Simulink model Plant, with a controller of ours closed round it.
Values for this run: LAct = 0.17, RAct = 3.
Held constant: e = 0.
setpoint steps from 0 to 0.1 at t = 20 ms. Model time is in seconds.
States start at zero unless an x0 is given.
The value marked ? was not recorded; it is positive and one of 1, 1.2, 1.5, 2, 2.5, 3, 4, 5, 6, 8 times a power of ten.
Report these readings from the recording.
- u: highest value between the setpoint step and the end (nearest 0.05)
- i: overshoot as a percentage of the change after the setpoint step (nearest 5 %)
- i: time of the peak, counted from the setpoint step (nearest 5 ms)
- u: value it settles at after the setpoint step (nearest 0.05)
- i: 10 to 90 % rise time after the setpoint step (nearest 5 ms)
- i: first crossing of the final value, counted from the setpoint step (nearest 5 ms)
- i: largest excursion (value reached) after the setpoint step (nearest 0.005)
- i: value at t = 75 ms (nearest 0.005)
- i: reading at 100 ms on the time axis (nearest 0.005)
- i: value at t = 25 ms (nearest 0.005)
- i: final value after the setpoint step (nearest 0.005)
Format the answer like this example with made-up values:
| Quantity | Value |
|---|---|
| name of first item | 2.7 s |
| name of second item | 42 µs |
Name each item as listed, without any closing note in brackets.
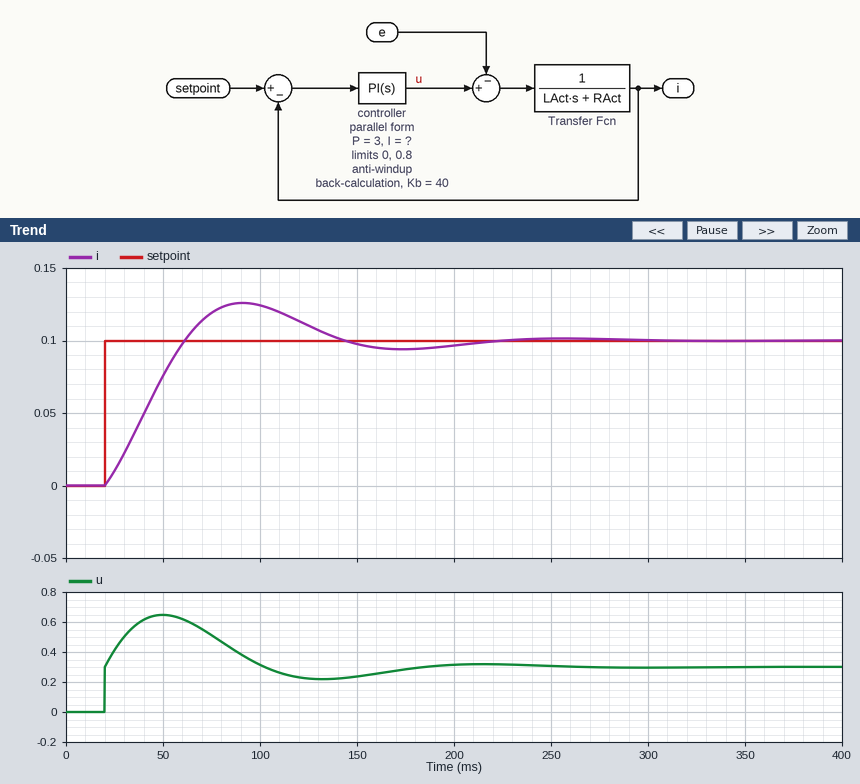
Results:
| Quantity | Value |
|---|---|
| u: highest value between the setpoint step and the end | 0.65 |
| i: overshoot as a percentage of the change after the setpoint step | 25 % |
| i: time of the peak, counted from the setpoint step | 70 ms |
| u: value it settles at after the setpoint step | 0.30 |
| i: 10 to 90 % rise time after the setpoint step | 30 ms |
| i: first crossing of the final value, counted from the setpoint step | 40 ms |
| i: largest excursion (value reached) after the setpoint step | 0.125 |
| i: value at t = 75 ms | 0.120 |
| i: reading at 100 ms on the time axis | 0.125 |
| i: value at t = 25 ms | 0.010 |
| i: final value after the setpoint step | 0.100 |
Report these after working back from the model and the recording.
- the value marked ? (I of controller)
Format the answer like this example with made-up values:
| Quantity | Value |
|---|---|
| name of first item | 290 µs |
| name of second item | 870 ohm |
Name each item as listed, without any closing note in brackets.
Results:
| Quantity | Value |
|---|---|
| the value marked ? | 300 |
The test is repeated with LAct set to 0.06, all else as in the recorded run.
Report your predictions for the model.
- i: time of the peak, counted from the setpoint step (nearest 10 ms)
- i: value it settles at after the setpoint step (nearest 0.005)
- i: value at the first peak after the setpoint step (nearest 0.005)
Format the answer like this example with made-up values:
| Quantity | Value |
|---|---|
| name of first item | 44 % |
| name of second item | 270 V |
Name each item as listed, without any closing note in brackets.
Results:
| Quantity | Value |
|---|---|
| i: time of the peak, counted from the setpoint step | 50 ms |
| i: value it settles at after the setpoint step | 0.100 |
| i: value at the first peak after the setpoint step | 0.105 |
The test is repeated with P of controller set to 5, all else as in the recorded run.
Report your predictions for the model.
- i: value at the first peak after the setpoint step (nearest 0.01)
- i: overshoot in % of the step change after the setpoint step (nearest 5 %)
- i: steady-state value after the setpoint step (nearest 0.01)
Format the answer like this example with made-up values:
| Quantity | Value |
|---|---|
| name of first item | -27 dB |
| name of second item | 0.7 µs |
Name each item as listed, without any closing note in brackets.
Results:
| Quantity | Value |
|---|---|
| i: value at the first peak after the setpoint step | 0.12 |
| i: overshoot in % of the step change after the setpoint step | 15 % |
| i: steady-state value after the setpoint step | 0.10 |
